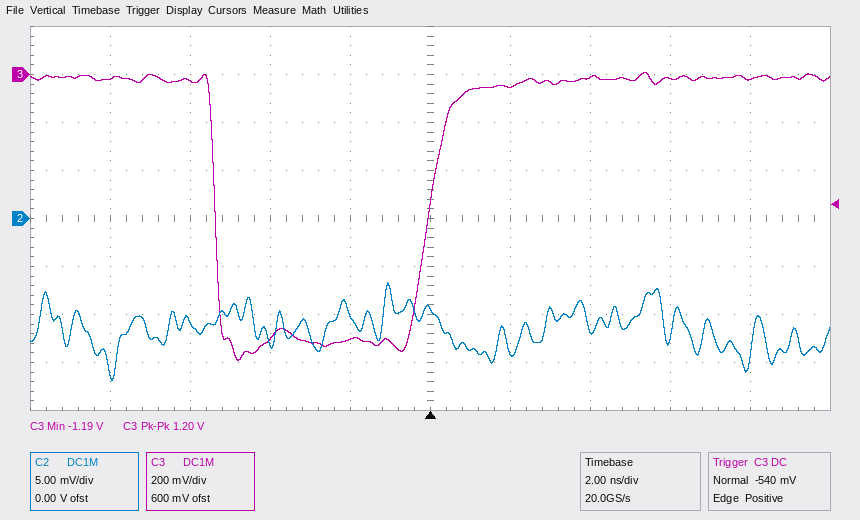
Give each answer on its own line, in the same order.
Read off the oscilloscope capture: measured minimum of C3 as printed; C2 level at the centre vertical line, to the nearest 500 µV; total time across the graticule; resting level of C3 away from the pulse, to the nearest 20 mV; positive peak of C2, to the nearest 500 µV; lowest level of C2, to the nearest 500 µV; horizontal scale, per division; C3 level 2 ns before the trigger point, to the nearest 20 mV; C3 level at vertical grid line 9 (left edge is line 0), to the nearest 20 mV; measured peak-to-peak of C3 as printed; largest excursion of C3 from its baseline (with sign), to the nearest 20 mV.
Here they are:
-1.19 V
-9.5 mV
20 ns
-20 mV
-6.5 mV
-17.0 mV
2 ns
-1.10 V
-20 mV
1.20 V
-1.18 V
